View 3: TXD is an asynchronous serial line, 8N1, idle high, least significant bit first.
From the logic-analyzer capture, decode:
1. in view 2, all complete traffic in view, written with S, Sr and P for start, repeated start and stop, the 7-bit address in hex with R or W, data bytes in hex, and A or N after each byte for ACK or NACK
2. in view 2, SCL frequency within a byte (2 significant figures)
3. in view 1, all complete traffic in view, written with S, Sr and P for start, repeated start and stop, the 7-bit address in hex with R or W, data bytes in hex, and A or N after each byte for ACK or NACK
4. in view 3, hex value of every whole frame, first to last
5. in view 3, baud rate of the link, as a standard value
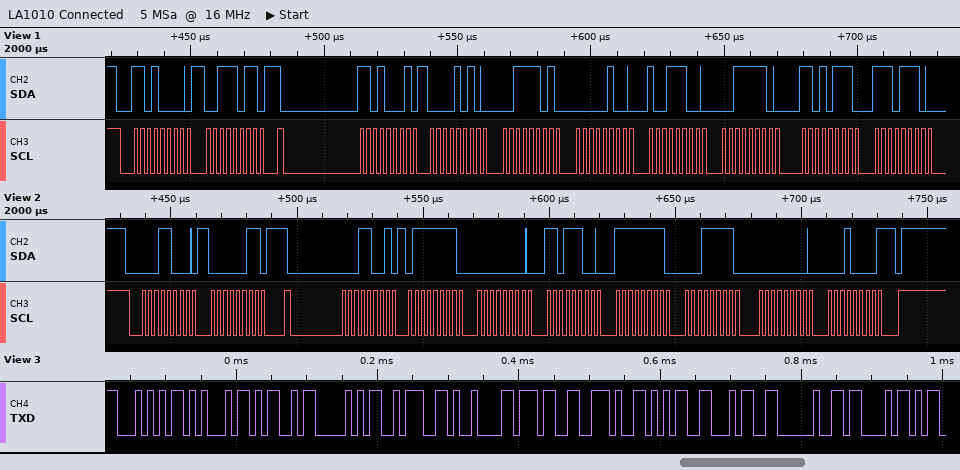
S 0CW A 03 A Sr 0CR A 7F A 00 A DC A FF A 1F A 00 A 10 N P
400 kHz
S 68W A 3B A Sr 68R A 0A A 3D A 04 A 9C A 3E A D7 A EE A
54 45 4D 50 3A 09 37 2E 35 34 20 43
115200 baud
